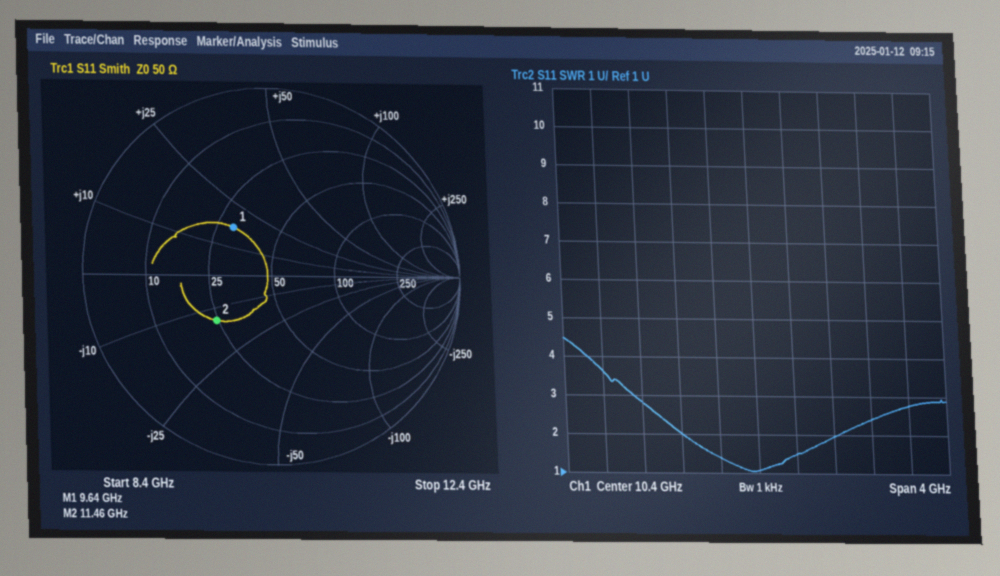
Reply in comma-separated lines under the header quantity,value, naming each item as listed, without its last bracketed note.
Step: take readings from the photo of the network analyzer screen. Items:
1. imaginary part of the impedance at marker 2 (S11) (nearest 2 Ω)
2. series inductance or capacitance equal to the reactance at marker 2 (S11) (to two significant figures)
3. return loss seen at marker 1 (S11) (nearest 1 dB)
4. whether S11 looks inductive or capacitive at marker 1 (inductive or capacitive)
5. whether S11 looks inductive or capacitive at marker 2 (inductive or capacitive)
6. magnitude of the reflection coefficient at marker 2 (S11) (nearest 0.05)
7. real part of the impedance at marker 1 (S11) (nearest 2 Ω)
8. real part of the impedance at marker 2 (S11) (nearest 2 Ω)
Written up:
quantity,value
imaginary part of the impedance at marker 2 (S11),-14 Ω
series inductance or capacitance equal to the reactance at marker 2 (S11),1.0 pF
return loss seen at marker 1 (S11),10 dB
whether S11 looks inductive or capacitive at marker 1,inductive
whether S11 looks inductive or capacitive at marker 2,capacitive
magnitude of the reflection coefficient at marker 2 (S11),0.40
real part of the impedance at marker 1 (S11),30 Ω
real part of the impedance at marker 2 (S11),24 Ω
